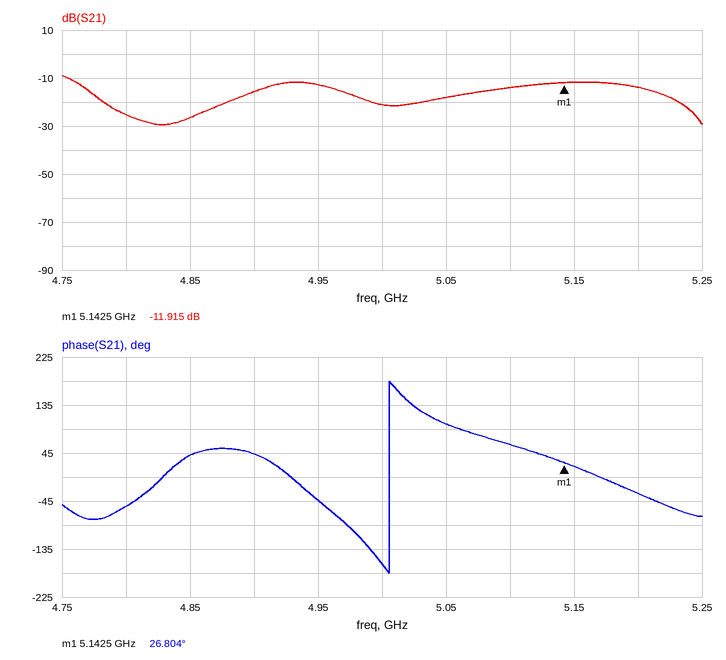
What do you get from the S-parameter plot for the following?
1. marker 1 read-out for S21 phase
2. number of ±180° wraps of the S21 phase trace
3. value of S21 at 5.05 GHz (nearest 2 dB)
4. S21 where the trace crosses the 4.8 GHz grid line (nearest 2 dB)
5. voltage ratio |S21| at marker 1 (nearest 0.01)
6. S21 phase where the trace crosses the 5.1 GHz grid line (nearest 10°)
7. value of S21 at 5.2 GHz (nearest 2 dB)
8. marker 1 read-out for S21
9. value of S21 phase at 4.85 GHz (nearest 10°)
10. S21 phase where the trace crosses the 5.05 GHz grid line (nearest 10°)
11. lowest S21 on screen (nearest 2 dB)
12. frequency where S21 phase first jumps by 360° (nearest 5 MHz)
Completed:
26.804°
1
-18 dB
-26 dB
0.25
60°
-14 dB
-11.915 dB
40°
100°
-30 dB
5.005 GHz
